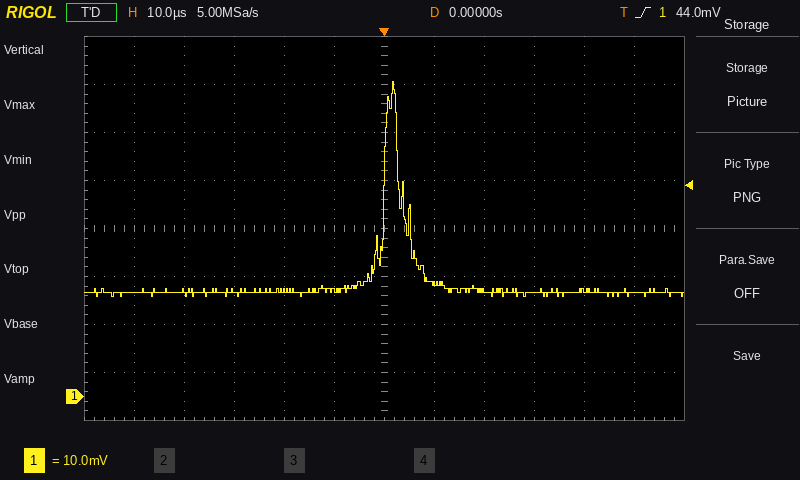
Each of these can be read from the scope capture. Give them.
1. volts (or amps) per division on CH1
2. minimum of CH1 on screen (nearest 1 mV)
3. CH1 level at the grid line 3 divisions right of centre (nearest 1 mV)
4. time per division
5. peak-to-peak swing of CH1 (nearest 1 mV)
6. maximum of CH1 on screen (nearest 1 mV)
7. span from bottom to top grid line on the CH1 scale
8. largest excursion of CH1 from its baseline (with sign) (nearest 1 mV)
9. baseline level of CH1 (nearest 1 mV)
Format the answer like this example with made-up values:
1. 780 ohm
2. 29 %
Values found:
1. 10 mV
2. 21 mV
3. 22 mV
4. 10 µs
5. 45 mV
6. 66 mV
7. 80 mV
8. +44 mV
9. 22 mV
